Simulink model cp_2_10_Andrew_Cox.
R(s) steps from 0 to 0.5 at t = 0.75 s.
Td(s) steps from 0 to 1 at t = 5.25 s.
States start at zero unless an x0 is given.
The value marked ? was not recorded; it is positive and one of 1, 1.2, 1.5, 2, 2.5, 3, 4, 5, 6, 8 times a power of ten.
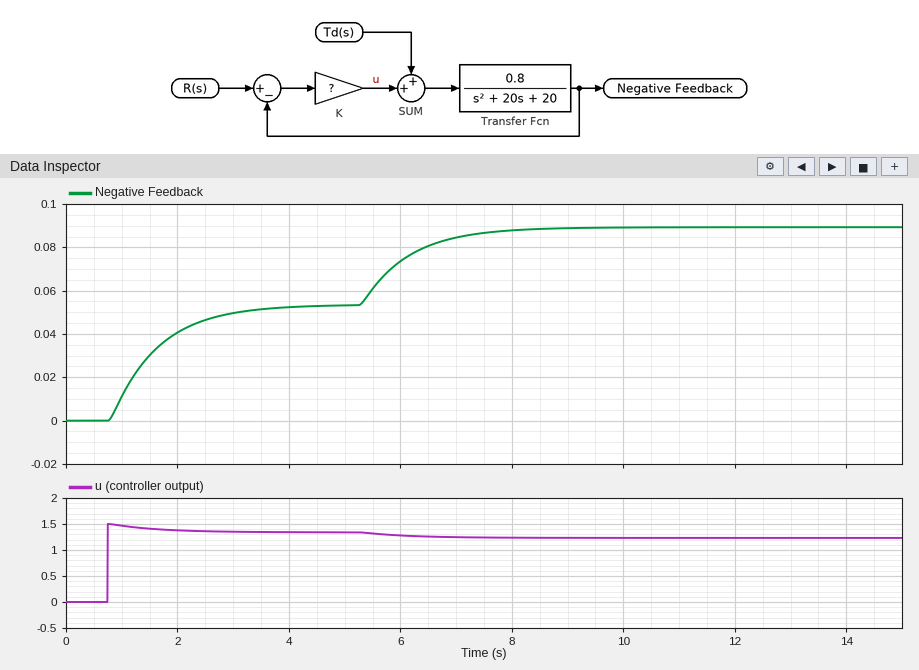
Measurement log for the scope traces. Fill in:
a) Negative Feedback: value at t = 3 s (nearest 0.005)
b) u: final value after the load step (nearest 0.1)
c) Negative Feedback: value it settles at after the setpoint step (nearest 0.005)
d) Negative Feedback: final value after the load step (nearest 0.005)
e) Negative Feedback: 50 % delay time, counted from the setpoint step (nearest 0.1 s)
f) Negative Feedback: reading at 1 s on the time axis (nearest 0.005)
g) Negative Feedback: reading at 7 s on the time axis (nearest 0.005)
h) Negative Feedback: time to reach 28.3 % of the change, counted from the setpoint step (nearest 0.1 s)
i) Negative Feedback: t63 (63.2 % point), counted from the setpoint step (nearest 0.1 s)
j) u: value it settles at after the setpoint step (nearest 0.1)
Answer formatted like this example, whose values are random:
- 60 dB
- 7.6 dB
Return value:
- 0.050
- 1.2
- 0.055
- 0.090
- 0.6 s
- 0.010
- 0.085
- 0.3 s
- 0.9 s
- 1.3
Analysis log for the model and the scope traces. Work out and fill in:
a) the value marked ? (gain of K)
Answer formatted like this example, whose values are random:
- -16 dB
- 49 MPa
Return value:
- 3
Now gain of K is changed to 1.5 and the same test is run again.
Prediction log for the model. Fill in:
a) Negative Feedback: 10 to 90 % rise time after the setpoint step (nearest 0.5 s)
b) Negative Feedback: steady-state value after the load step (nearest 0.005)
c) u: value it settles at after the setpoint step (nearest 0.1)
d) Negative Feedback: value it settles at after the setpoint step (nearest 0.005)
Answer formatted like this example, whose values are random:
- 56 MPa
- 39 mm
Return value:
- 2.0 s
- 0.065
- 0.7
- 0.030
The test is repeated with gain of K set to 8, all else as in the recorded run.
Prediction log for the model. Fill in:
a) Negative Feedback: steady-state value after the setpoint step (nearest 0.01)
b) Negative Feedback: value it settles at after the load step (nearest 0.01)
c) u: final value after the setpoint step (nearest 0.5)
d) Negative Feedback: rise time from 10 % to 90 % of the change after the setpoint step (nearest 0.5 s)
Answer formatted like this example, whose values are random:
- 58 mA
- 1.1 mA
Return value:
- 0.12
- 0.15
- 3.0
- 1.5 s
